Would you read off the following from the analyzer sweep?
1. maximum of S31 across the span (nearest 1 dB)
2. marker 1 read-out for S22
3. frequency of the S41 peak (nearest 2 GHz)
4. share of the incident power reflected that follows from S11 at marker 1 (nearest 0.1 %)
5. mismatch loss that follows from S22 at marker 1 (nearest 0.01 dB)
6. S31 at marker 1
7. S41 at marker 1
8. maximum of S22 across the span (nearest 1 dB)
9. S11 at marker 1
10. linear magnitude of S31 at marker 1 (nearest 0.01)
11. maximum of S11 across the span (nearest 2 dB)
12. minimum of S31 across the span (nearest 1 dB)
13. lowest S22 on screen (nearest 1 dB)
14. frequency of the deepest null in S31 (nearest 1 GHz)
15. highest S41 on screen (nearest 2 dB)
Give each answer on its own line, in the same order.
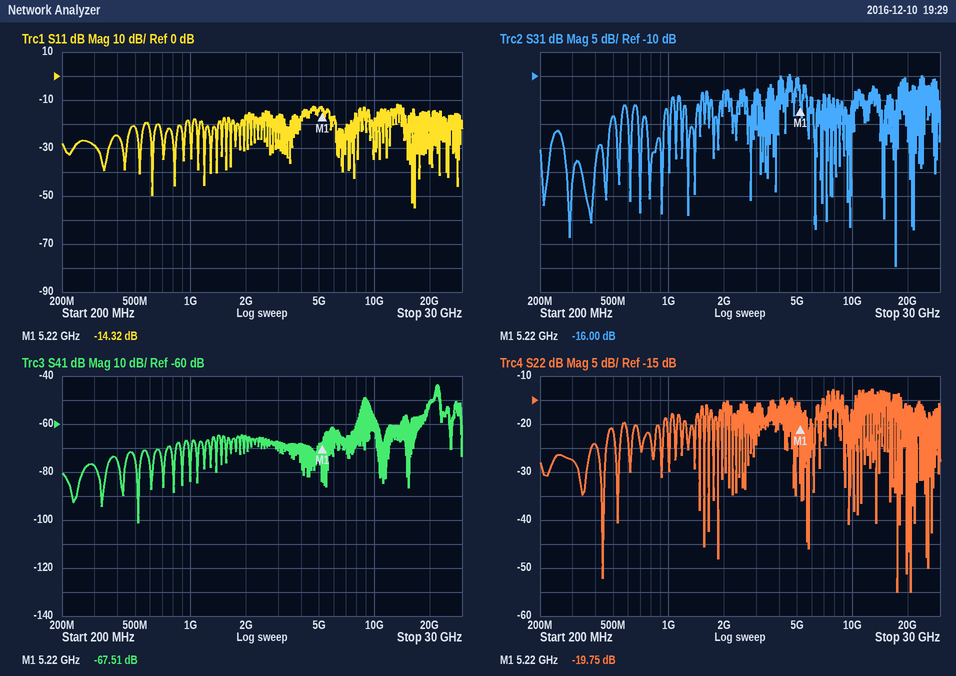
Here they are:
-10 dB
-19.75 dB
22 GHz
3.7 %
0.05 dB
-16.00 dB
-67.51 dB
-13 dB
-14.32 dB
0.16
-12 dB
-50 dB
-55 dB
17 GHz
-44 dB
